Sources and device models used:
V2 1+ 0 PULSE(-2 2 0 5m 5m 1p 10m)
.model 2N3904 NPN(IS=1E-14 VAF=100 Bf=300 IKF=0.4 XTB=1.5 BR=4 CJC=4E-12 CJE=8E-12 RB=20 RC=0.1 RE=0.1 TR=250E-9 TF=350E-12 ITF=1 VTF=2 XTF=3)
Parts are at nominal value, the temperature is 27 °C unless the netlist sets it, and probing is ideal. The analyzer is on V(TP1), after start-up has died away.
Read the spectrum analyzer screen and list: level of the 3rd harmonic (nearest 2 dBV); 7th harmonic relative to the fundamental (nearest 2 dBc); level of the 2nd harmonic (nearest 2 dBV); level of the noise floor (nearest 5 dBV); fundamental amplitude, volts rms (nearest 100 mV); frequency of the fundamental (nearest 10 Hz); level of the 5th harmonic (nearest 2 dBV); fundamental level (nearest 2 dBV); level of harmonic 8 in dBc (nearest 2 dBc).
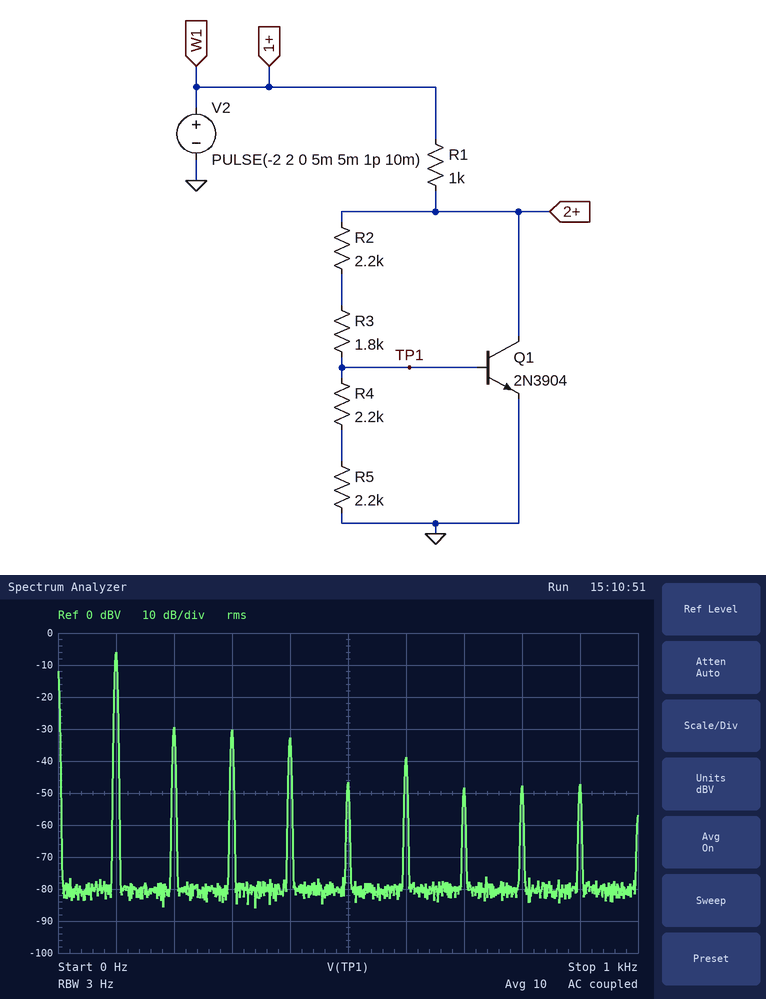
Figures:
-30 dBV
-42 dBc
-30 dBV
-80 dBV
500 mV
100 Hz
-46 dBV
-6 dBV
-42 dBc
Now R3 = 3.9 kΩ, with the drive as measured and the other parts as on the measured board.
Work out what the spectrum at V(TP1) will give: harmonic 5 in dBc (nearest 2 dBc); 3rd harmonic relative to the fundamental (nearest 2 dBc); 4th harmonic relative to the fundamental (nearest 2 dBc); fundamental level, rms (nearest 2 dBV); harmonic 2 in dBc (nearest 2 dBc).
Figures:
-30 dBc
-20 dBc
-30 dBc
-8 dBV
-26 dBc
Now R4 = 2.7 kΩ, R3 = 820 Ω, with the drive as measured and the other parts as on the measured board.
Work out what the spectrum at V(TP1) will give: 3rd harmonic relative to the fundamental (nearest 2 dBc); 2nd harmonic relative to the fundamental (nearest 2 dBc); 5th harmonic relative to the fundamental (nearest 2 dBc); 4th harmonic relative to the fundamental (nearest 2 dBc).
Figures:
-28 dBc
-20 dBc
-42 dBc
-24 dBc
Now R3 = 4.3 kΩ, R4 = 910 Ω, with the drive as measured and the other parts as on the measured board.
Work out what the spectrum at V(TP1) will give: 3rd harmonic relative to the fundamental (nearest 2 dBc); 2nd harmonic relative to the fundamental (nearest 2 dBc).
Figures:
-18 dBc
-28 dBc
